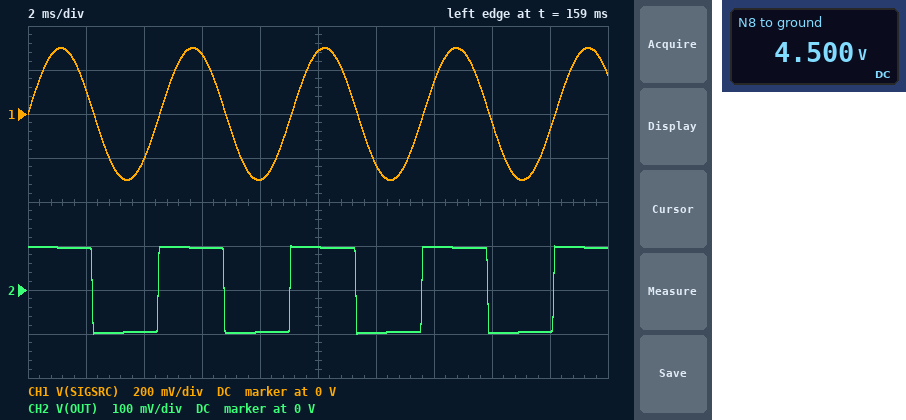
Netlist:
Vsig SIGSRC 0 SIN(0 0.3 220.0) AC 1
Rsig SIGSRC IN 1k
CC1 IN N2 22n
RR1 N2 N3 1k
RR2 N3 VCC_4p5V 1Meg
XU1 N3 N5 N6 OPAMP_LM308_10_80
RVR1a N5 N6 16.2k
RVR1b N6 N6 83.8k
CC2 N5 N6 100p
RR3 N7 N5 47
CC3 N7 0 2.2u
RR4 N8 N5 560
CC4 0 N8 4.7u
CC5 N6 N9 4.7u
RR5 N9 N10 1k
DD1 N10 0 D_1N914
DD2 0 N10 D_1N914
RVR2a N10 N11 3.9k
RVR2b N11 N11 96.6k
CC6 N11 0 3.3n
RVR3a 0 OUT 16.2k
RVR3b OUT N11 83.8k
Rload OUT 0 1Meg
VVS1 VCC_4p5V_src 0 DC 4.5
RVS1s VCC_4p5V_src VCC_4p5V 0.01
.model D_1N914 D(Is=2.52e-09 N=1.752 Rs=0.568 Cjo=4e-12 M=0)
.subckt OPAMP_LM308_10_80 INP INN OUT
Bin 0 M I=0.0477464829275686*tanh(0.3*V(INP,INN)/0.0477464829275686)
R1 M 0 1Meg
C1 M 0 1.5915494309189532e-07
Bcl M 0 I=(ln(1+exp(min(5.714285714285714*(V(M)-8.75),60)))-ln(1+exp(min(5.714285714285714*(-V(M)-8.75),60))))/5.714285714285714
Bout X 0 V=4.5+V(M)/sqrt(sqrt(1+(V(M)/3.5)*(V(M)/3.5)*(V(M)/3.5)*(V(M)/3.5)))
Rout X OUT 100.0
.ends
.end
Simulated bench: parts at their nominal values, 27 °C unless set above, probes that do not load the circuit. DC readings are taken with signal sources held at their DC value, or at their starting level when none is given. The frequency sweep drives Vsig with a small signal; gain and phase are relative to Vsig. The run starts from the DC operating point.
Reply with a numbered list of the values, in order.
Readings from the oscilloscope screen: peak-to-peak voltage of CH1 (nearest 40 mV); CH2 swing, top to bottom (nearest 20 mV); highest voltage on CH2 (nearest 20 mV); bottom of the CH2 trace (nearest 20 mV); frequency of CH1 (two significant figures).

1. 600 mV
2. 200 mV
3. 100 mV
4. -100 mV
5. 220 Hz
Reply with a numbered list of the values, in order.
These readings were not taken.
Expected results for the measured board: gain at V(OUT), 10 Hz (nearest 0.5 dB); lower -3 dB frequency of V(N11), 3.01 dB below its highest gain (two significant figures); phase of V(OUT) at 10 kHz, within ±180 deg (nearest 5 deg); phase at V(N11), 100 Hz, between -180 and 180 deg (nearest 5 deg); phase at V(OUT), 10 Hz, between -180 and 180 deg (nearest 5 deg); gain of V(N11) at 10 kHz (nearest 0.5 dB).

1. -1.0 dB
2. 720 Hz
3. -130 deg
4. 60 deg
5. 115 deg
6. 26.0 dB
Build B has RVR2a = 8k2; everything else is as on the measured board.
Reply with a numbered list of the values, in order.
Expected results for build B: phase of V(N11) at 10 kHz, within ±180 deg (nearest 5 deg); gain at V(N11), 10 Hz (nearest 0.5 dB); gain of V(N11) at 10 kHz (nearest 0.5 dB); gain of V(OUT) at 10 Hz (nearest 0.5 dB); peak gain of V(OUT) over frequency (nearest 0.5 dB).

1. -145 deg
2. 14.5 dB
3. 22.5 dB
4. -1.5 dB
5. 33.5 dB
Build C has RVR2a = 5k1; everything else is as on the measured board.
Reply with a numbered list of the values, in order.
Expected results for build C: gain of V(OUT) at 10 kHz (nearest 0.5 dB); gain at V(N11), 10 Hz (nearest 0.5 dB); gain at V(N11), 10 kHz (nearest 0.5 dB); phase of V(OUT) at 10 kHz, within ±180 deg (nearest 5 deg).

1. 9.0 dB
2. 14.5 dB
3. 25.0 dB
4. -135 deg
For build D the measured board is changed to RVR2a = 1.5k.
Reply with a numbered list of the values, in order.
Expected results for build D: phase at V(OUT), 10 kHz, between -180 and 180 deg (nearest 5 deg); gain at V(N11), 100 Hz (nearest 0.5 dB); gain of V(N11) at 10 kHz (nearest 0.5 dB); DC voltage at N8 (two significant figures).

1. -115 deg
2. 32.5 dB
3. 28.0 dB
4. 4.5 V
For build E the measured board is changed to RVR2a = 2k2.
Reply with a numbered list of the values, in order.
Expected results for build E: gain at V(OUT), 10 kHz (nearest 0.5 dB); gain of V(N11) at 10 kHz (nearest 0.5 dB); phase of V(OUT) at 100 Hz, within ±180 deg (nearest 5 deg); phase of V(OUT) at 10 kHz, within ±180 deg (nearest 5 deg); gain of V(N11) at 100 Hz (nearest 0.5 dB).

1. 11.5 dB
2. 27.5 dB
3. 60 deg
4. -120 deg
5. 32.5 dB
